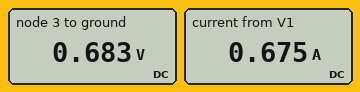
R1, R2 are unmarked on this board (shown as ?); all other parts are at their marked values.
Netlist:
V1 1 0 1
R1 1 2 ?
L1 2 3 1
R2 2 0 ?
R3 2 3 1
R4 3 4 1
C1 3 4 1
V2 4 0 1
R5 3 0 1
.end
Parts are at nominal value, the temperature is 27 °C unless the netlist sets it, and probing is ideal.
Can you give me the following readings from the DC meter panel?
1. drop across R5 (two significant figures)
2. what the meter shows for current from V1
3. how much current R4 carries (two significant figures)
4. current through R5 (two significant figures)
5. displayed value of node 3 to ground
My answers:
680 mV
0.675 A
320 mA
680 mA
0.683 V
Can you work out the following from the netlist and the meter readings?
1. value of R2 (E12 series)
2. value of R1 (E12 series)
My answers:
2.2 Ω
0.47 Ω
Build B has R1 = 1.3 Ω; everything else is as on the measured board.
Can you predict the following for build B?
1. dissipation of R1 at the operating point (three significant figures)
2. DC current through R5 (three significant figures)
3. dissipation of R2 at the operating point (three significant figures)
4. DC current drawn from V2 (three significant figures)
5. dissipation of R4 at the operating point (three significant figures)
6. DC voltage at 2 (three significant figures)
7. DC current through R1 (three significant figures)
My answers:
157 mW
549 mA
137 mW
451 mA
204 mW
549 mV
347 mA
